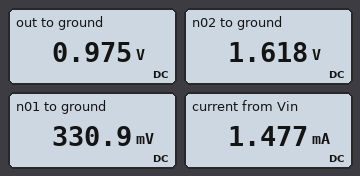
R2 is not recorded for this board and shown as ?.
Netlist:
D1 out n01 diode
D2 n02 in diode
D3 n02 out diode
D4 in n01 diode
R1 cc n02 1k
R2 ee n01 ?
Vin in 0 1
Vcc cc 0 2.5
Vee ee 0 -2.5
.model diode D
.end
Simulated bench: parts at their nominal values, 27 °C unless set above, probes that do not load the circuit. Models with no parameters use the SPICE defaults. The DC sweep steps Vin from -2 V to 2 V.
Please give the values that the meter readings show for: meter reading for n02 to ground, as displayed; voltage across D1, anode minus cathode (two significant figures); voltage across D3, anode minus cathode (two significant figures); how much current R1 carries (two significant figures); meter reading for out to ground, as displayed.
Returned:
1.618 V
640 mV
640 mV
880 µA
0.975 V
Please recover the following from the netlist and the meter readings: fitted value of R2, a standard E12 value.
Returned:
1.2 kΩ
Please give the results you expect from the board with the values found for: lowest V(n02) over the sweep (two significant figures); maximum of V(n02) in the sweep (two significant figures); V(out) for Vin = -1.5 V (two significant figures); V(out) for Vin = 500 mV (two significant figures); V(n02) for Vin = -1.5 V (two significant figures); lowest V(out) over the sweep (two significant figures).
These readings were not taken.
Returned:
-1.3 V
2.5 V
-1.4 V
490 mV
-820 mV
-1.9 V
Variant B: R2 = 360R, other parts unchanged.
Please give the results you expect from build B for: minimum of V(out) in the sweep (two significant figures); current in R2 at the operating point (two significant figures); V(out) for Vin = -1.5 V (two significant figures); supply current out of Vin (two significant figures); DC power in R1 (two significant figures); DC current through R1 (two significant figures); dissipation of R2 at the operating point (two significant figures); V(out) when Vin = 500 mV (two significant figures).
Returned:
-1.9 V
7.8 mA
-1.5 V
6.9 mA
820 µW
910 µA
22 mW
460 mV
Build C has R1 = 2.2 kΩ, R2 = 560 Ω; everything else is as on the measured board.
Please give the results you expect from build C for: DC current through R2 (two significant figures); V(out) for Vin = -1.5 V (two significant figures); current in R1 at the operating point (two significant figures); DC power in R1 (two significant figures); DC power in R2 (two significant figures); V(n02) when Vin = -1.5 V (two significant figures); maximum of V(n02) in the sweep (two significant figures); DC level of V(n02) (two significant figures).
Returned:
5.0 mA
-1.5 V
420 µA
400 µW
14 mW
-840 mV
2.4 V
1.6 V
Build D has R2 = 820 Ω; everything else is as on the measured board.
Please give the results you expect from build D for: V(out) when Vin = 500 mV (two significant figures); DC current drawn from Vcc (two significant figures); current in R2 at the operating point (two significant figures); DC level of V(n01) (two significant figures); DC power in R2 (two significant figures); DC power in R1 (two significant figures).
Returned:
480 mV
890 µA
3.4 mA
320 mV
9.7 mW
790 µW
